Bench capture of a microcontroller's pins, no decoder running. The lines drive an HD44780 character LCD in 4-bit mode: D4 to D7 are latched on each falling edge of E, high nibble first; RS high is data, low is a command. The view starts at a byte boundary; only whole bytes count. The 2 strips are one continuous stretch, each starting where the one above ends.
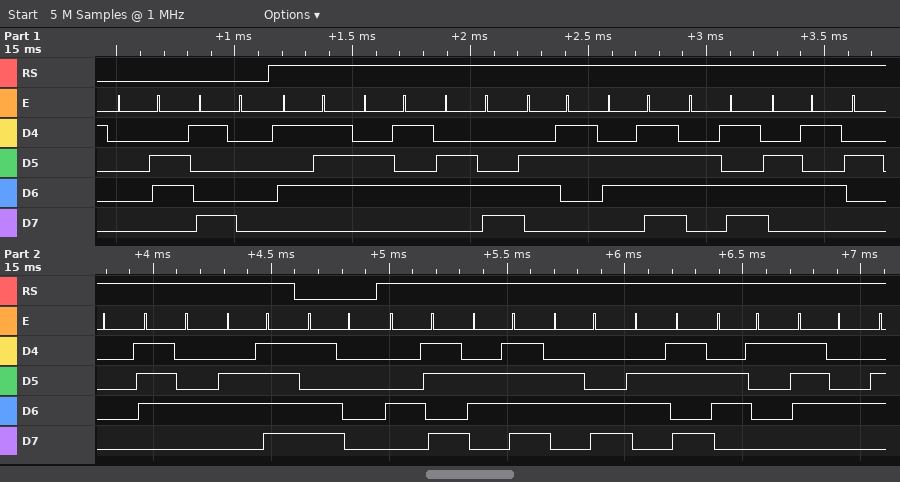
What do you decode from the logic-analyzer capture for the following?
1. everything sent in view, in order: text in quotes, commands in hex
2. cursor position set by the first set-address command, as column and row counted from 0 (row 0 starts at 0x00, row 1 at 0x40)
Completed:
0x06 0x90 "Welcome to" 0xD0 "Kolkat"
column 16, row 0
